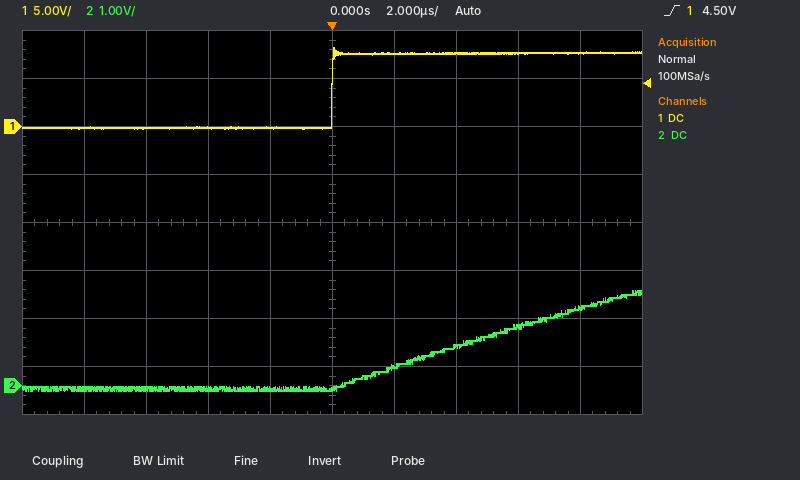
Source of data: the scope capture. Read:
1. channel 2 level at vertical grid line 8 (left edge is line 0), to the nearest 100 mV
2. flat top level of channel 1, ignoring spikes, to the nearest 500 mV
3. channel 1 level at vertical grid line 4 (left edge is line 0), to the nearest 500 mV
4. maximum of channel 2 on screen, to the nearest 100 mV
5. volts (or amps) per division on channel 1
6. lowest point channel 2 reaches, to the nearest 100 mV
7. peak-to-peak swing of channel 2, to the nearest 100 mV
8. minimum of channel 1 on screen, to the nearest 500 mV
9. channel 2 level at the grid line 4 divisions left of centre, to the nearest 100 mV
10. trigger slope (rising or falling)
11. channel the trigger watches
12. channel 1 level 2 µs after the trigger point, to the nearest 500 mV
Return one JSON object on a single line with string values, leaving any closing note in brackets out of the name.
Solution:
{"channel 2 level at vertical grid line 8 (left edge is line 0), to the nearest 100 mV": "1.2 V", "flat top level of channel 1, ignoring spikes, to the nearest 500 mV": "7.5 V", "channel 1 level at vertical grid line 4 (left edge is line 0), to the nearest 500 mV": "0.0 V", "maximum of channel 2 on screen, to the nearest 100 mV": "2.0 V", "volts (or amps) per division on channel 1": "5 V", "lowest point channel 2 reaches, to the nearest 100 mV": "-100 mV", "peak-to-peak swing of channel 2, to the nearest 100 mV": "2.1 V", "minimum of channel 1 on screen, to the nearest 500 mV": "0.0 V", "channel 2 level at the grid line 4 divisions left of centre, to the nearest 100 mV": "-100 mV", "trigger slope": "rising", "channel the trigger watches": "channel 1", "channel 1 level 2 µs after the trigger point, to the nearest 500 mV": "7.5 V"}
